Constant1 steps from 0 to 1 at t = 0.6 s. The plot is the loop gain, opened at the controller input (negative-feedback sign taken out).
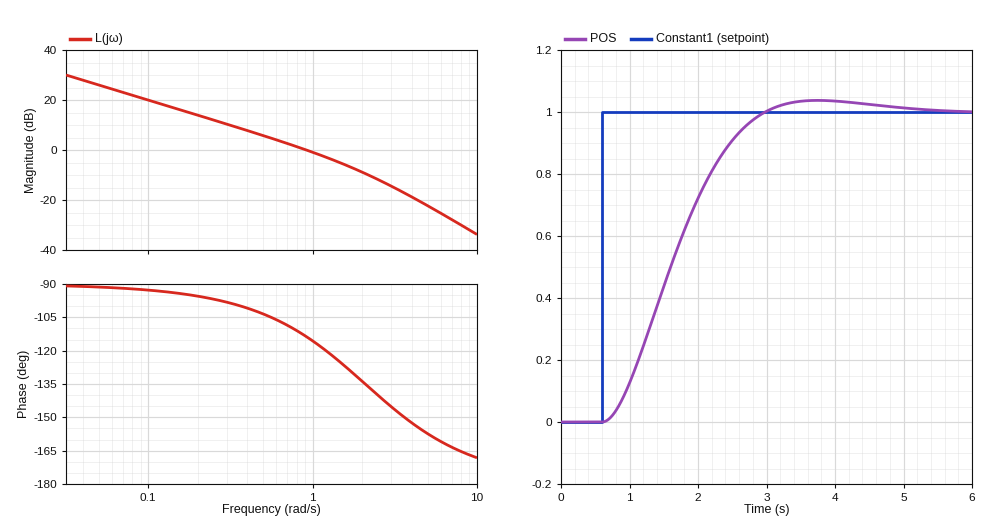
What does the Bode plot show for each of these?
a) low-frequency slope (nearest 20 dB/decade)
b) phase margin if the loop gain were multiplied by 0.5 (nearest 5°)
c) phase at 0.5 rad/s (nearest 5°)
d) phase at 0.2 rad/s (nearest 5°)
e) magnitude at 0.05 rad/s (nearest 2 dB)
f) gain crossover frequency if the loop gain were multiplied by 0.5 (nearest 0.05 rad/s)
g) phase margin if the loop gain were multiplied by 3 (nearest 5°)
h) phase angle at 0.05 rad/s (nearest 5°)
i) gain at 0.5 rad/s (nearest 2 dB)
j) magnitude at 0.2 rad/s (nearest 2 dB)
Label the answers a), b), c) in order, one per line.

a) -20 dB/decade
b) 75°
c) -105°
d) -95°
e) 26 dB
f) 0.50 rad/s
g) 45°
h) -90°
i) 6 dB
j) 14 dB
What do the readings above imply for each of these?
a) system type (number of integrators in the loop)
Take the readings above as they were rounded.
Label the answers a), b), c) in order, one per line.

a) 1
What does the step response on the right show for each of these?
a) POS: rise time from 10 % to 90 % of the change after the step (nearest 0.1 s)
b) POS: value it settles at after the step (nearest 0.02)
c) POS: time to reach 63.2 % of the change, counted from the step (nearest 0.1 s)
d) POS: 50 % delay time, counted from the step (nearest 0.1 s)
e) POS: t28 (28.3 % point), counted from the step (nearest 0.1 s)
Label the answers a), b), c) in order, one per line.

a) 1.5 s
b) 1.00
c) 1.2 s
d) 1.0 s
e) 0.7 s
